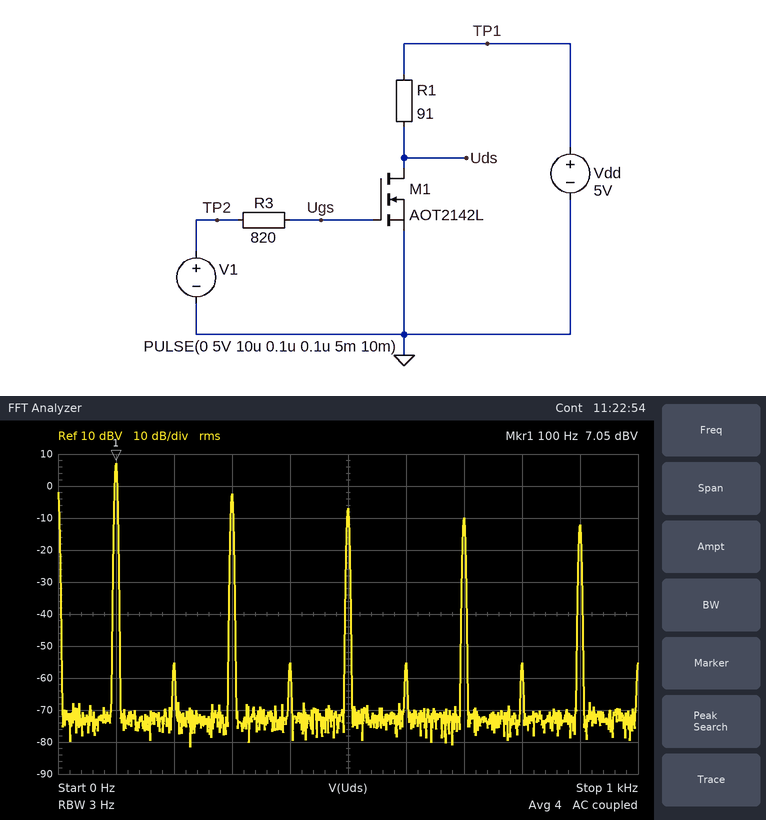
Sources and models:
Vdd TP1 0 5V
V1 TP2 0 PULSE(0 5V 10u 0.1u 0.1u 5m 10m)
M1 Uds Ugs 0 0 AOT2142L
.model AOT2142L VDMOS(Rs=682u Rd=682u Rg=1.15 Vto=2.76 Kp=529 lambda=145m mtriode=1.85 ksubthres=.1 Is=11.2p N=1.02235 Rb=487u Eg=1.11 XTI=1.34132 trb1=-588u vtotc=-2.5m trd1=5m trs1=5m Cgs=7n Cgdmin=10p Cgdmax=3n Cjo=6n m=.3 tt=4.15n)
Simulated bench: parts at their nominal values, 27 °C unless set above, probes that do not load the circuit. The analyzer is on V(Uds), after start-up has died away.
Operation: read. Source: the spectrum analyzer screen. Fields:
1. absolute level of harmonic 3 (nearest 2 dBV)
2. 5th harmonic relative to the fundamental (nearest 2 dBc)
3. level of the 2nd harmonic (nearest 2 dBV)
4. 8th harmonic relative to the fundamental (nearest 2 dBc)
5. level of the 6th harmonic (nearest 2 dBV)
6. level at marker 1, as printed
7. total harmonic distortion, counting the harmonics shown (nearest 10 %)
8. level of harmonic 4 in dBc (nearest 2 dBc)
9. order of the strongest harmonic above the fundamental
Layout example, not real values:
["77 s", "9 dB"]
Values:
["-2 dBV", "-14 dBc", "-56 dBV", "-62 dBc", "-56 dBV", "7.05 dBV", "40 %", "-62 dBc", "3"]
